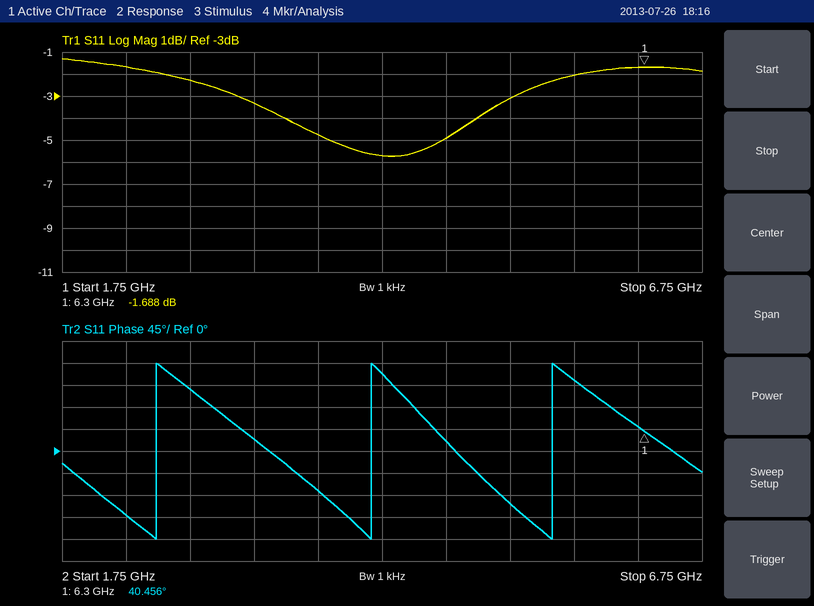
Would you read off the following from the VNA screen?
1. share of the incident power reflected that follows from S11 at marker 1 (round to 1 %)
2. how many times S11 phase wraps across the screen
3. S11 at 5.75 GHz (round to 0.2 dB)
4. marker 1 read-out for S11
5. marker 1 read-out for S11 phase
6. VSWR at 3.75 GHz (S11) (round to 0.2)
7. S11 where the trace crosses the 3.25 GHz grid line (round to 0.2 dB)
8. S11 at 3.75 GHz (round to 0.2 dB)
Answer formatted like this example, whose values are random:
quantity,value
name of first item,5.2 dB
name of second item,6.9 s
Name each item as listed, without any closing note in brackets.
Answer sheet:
quantity,value
share of the incident power reflected that follows from S11 at marker 1,68 %
how many times S11 phase wraps across the screen,3
S11 at 5.75 GHz,-2.0 dB
marker 1 read-out for S11,-1.688 dB
marker 1 read-out for S11 phase,40.456°
VSWR at 3.75 GHz (S11),3.8
S11 where the trace crosses the 3.25 GHz grid line,-3.4 dB
S11 at 3.75 GHz,-4.8 dB
